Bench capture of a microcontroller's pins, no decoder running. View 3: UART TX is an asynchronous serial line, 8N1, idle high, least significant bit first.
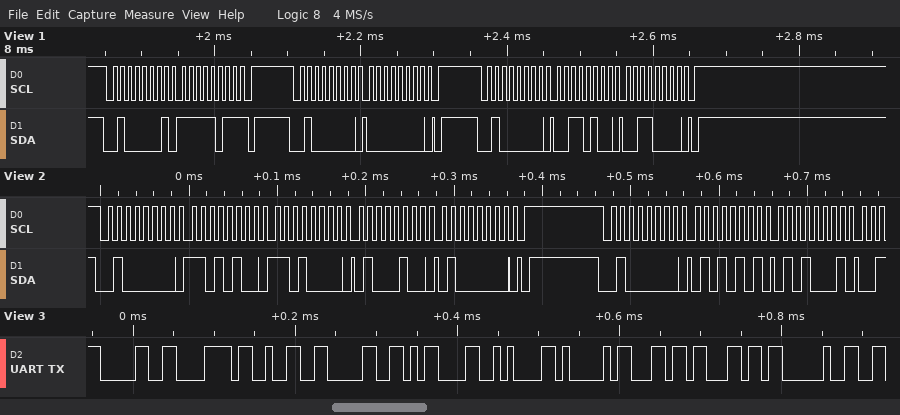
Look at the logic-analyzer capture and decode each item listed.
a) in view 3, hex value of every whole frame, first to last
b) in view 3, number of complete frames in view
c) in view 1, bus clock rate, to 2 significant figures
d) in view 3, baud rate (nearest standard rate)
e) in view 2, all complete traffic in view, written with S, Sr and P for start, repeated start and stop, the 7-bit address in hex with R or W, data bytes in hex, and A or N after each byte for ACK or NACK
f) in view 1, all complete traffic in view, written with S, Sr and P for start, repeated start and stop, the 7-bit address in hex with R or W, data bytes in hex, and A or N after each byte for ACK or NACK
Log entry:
0x30 0x78 0x32 0x30 0x0D 0x0A 0x41 0x6C 0x6C 0x20
10
100 kHz
115200 baud
S 20W A D4 A D0 A 44 A 40 A P S 20W A 55 A 51 A
S 20R A FB N P S 20W A 00 A P S 20W A 34 A 30 A P
